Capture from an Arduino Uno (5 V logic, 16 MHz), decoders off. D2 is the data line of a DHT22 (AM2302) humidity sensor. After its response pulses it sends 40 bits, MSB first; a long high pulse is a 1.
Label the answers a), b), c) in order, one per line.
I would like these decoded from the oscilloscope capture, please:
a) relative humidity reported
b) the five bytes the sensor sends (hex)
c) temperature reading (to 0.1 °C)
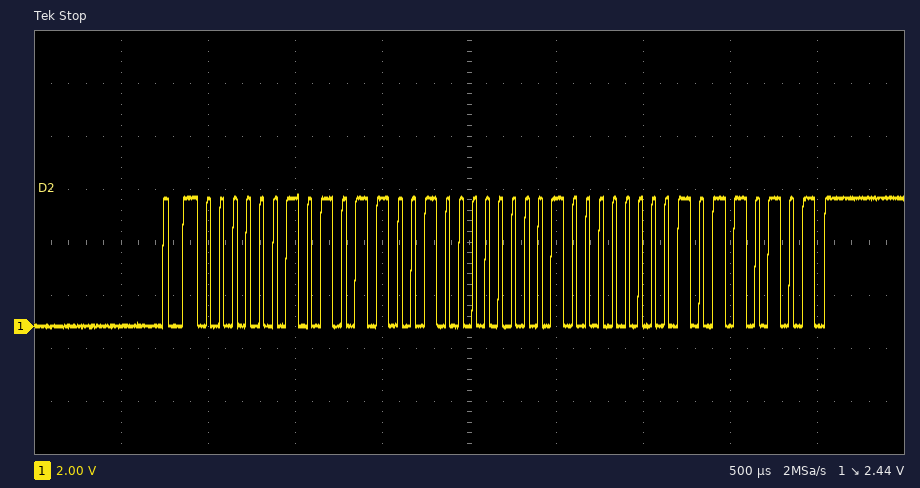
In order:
a) 69.0 %
b) 02 B2 01 00 B5
c) 25.6 °C
